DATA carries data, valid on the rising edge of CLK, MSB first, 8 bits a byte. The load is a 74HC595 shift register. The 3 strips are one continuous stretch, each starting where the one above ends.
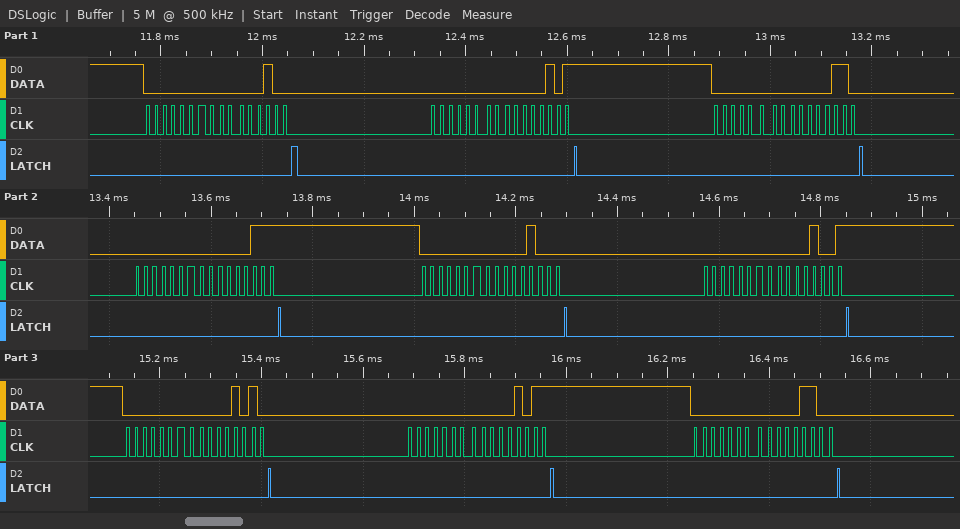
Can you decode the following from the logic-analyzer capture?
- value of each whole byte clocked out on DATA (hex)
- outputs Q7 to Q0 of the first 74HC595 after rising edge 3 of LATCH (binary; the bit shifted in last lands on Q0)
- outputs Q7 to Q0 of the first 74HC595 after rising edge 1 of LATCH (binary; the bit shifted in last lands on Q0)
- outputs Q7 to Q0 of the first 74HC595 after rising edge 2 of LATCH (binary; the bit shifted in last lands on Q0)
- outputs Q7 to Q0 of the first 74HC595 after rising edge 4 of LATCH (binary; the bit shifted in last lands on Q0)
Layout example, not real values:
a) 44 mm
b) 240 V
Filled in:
a) 00 04 00 05 00 06 00 07 00 08 00 09 00 0A 00 0B 00 0C
b) 00000110
c) 00000100
d) 00000101
e) 00000111
